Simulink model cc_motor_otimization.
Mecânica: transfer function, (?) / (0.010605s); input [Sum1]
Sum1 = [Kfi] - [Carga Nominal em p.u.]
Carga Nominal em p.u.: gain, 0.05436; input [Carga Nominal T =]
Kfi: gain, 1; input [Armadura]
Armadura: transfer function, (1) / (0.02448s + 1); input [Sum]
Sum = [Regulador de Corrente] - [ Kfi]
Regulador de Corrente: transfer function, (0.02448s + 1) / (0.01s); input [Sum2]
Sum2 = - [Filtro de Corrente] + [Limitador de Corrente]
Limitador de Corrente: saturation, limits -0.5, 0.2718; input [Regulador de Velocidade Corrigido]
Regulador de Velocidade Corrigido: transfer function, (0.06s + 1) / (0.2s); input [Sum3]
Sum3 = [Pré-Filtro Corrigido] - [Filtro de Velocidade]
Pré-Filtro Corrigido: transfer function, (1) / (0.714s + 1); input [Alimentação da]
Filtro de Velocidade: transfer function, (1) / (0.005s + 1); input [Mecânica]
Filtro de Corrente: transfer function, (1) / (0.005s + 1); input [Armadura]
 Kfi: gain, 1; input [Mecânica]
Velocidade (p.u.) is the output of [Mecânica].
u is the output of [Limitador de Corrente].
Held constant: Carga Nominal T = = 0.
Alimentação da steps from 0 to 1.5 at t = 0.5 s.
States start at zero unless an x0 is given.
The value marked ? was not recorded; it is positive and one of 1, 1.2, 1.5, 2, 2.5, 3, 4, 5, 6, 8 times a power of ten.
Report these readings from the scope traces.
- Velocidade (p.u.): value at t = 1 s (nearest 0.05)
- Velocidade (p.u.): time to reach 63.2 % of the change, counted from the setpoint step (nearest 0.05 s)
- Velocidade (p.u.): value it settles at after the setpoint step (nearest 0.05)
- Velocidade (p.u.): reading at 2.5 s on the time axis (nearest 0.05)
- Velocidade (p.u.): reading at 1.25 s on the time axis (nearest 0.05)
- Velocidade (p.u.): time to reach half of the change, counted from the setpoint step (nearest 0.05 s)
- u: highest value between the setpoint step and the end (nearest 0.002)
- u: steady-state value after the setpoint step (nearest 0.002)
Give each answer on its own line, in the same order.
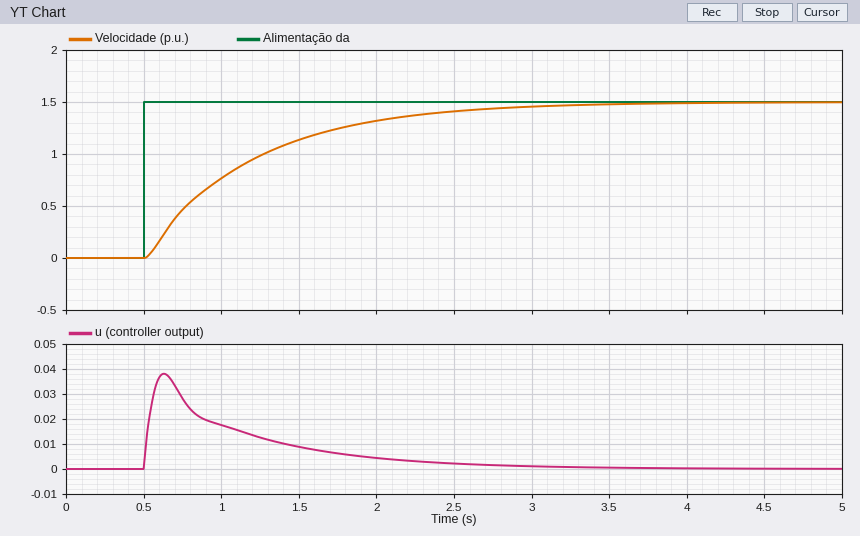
0.75
0.70 s
1.50
1.40
1.00
0.50 s
0.038
0.000
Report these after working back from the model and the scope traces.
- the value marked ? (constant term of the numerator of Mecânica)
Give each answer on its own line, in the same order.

1.5
